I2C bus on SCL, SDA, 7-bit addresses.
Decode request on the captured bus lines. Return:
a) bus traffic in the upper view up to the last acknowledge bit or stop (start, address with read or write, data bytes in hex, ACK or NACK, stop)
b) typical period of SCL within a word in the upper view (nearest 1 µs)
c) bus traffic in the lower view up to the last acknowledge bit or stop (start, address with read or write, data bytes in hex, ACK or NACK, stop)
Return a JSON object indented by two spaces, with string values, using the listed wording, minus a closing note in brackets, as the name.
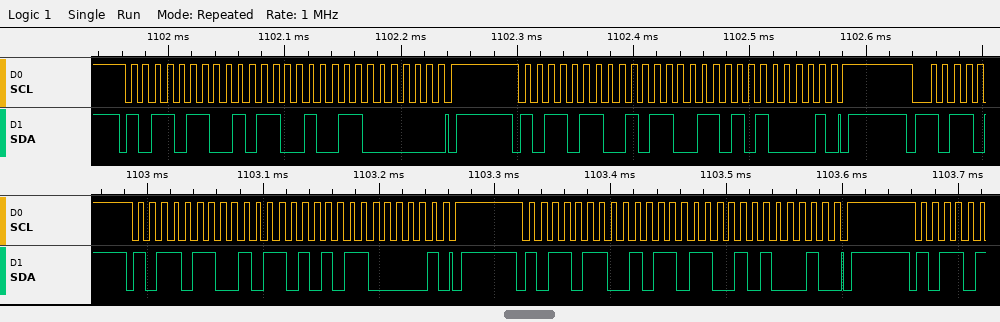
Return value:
{
  "bus traffic in the upper view up to the last acknowledge bit or stop": "start, address 5B write ACK, B2 ACK, C0 ACK, stop, start, address 5B write ACK, B3 ACK, A1 ACK, stop",
  "typical period of SCL within a word in the upper view": "10 µs",
  "bus traffic in the lower view up to the last acknowledge bit or stop": "start, address 5B write ACK, B5 ACK, C1 ACK, stop, start, address 5B write ACK, B6 ACK, A2 ACK, stop"
}
